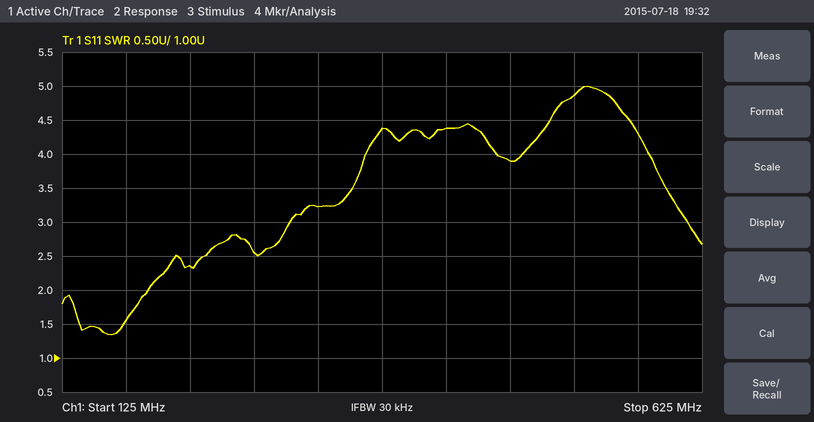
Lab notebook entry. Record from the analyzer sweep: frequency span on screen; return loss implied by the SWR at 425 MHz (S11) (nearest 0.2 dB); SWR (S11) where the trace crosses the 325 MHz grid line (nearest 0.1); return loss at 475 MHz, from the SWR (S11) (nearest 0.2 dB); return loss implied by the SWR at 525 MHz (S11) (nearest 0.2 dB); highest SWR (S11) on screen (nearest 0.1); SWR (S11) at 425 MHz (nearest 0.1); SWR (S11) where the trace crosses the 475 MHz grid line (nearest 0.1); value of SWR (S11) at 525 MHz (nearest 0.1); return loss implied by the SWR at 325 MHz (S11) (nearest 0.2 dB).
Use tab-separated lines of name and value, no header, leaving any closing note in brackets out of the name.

frequency span on screen	500 MHz
return loss implied by the SWR at 425 MHz (S11)	4.0 dB
SWR (S11) where the trace crosses the 325 MHz grid line	3.2
return loss at 475 MHz, from the SWR (S11)	4.6 dB
return loss implied by the SWR at 525 MHz (S11)	3.6 dB
highest SWR (S11) on screen	5.0
SWR (S11) at 425 MHz	4.4
SWR (S11) where the trace crosses the 475 MHz grid line	3.9
value of SWR (S11) at 525 MHz	4.9
return loss implied by the SWR at 325 MHz (S11)	5.6 dB
